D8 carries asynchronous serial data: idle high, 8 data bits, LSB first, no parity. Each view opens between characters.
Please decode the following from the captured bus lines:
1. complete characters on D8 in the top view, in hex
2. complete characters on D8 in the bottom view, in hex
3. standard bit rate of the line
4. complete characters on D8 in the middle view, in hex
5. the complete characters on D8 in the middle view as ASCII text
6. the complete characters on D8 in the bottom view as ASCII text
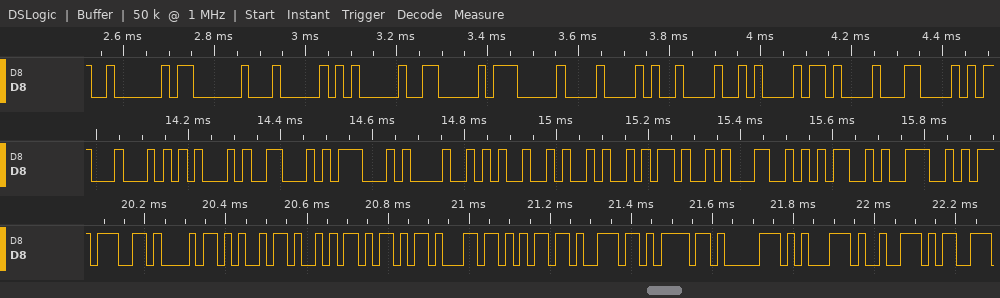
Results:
02, 03, 04, 05, 06, 07, 08, 09, 0A, 0B, 0C
67, 68, 69, 6A, 6B, 6C, 6D, 6E, 6F, 70, 71, 72
57600 baud
44, 45, 46, 47, 48, 49, 4A, 4B, 4C, 4D, 4E
"DEFGHIJKLMN"
"ghijklmnopqr"
